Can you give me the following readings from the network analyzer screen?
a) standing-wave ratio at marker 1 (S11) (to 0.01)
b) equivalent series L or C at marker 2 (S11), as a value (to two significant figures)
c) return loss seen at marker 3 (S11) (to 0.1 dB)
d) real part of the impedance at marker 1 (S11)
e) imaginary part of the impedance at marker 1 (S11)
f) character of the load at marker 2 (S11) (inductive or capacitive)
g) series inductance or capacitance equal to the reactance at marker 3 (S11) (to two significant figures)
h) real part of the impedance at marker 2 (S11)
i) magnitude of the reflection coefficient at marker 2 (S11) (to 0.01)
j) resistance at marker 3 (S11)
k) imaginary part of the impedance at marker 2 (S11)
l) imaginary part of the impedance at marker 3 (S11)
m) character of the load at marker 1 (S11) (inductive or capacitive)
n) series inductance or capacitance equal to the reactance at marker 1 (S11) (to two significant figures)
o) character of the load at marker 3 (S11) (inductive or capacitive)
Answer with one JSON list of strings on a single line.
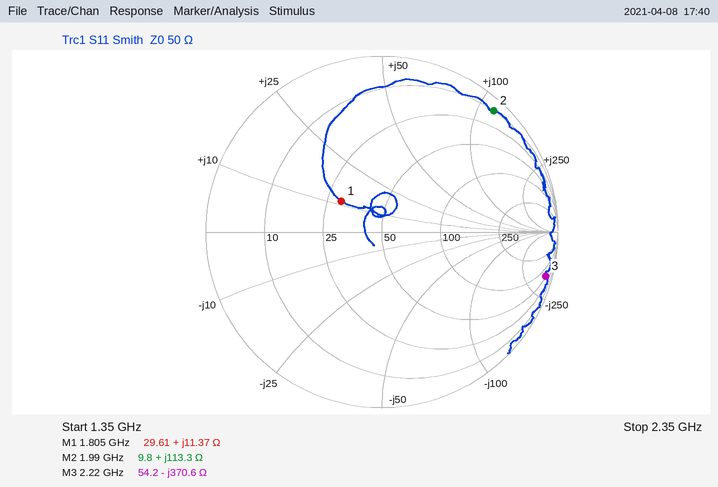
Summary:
["1.82", "9.1 nH", "0.3 dB", "29.61 Ω", "+11.37 Ω", "inductive", "190 fF", "9.8 Ω", "0.94", "54.2 Ω", "+113.3 Ω", "-370.6 Ω", "inductive", "1.0 nH", "capacitive"]
